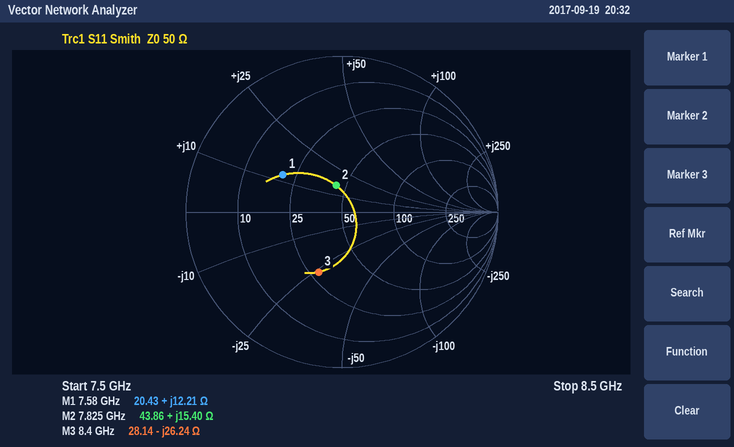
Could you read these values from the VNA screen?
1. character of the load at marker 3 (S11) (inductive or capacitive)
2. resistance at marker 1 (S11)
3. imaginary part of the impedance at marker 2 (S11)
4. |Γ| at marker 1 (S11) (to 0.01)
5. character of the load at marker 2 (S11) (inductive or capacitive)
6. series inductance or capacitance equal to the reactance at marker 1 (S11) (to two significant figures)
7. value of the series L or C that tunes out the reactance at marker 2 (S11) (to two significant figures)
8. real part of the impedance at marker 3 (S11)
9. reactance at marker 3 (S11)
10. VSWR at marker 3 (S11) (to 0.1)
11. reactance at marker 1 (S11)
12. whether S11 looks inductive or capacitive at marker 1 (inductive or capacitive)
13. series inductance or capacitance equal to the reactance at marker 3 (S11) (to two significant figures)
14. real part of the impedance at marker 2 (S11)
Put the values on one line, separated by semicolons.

capacitive; 20.43 Ω; +15.40 Ω; 0.45; inductive; 260 pH; 1.3 pF; 28.14 Ω; -26.24 Ω; 2.4; +12.21 Ω; inductive; 720 fF; 43.86 Ω
